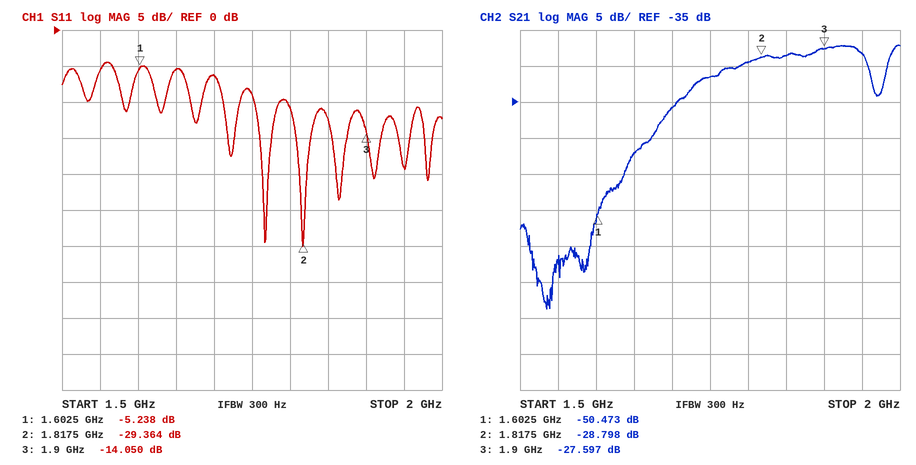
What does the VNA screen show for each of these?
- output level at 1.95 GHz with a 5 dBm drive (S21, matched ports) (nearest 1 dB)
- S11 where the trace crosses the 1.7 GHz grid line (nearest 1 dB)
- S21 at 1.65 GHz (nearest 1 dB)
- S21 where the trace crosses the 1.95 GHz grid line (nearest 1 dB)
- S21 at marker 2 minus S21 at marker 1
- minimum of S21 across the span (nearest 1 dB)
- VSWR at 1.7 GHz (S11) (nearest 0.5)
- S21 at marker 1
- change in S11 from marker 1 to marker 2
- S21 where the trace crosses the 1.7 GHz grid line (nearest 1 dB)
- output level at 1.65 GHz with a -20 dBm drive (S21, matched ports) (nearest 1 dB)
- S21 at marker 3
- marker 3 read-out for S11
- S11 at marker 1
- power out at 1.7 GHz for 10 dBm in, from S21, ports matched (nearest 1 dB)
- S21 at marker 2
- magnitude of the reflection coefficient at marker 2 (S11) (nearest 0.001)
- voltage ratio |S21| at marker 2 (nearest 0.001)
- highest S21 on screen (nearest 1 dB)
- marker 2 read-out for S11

-23 dBm
-6 dB
-42 dB
-28 dB
21.675 dB
-64 dB
3.0
-50.473 dB
-24.126 dB
-36 dB
-62 dBm
-27.597 dB
-14.050 dB
-5.238 dB
-26 dBm
-28.798 dB
0.034
0.036
-27 dB
-29.364 dB
